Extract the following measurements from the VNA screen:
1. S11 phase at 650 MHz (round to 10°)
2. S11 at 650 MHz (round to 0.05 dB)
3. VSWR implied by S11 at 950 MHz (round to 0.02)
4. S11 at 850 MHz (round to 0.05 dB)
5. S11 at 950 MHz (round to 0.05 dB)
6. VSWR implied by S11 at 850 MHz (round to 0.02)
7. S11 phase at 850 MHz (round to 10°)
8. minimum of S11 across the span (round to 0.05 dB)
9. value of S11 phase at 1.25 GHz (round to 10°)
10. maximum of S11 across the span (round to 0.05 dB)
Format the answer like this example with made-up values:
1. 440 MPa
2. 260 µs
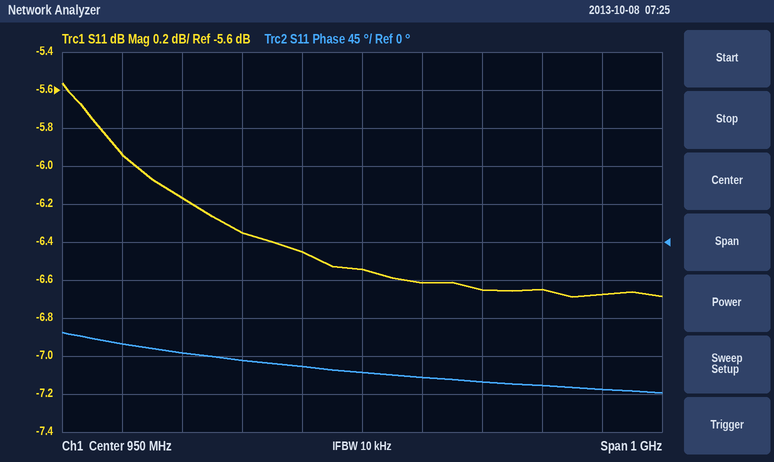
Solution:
1. -130°
2. -6.15 dB
3. 2.78
4. -6.45 dB
5. -6.55 dB
6. 2.82
7. -150°
8. -6.70 dB
9. -170°
10. -5.55 dB
